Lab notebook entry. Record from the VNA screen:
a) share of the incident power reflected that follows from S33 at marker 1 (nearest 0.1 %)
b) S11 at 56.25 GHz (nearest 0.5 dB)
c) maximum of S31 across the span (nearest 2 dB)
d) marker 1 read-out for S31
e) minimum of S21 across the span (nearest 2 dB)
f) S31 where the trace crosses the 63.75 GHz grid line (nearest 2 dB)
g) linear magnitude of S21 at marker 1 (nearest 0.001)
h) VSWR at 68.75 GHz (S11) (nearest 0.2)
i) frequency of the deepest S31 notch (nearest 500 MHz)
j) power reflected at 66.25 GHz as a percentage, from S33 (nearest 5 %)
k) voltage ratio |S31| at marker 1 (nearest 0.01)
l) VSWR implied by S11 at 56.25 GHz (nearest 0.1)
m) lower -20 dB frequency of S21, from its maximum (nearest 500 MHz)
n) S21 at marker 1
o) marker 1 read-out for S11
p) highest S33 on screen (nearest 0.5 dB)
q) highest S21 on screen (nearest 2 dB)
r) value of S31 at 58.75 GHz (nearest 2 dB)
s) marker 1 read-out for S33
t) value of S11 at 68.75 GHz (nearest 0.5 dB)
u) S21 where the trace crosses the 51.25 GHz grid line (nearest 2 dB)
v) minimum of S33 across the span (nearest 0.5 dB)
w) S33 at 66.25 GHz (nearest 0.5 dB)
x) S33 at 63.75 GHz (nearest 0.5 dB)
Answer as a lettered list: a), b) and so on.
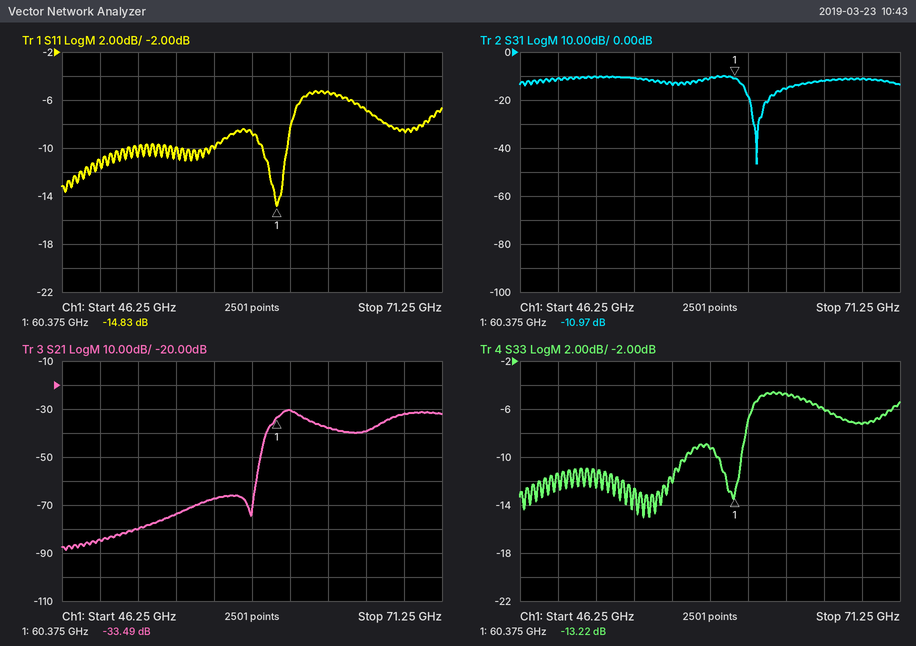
a) 4.8 %
b) -10.0 dB
c) -10 dB
d) -10.97 dB
e) -88 dB
f) -16 dB
g) 0.021
h) 2.2
i) 62.0 GHz
j) 25 %
k) 0.28
l) 1.9
m) 59.5 GHz
n) -33.49 dB
o) -14.83 dB
p) -4.5 dB
q) -30 dB
r) -10 dB
s) -13.22 dB
t) -8.5 dB
u) -80 dB
v) -15.0 dB
w) -6.0 dB
x) -4.5 dB
